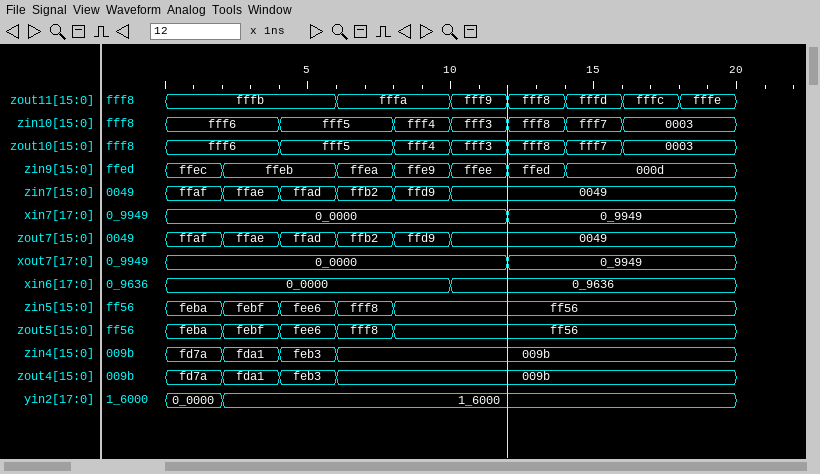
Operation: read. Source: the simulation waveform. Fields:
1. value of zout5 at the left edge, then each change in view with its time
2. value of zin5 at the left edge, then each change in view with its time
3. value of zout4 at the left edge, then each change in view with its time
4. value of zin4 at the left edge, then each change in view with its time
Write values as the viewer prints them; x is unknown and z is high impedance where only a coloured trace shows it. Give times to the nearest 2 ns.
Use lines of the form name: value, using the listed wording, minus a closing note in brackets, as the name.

value of zout5 at the left edge, then each change in view with its time: feba, febf at 2 ns, fee6 at 4 ns, fff8 at 6 ns, ff56 at 8 ns
value of zin5 at the left edge, then each change in view with its time: feba, febf at 2 ns, fee6 at 4 ns, fff8 at 6 ns, ff56 at 8 ns
value of zout4 at the left edge, then each change in view with its time: fd7a, fda1 at 2 ns, feb3 at 4 ns, 009b at 6 ns
value of zin4 at the left edge, then each change in view with its time: fd7a, fda1 at 2 ns, feb3 at 4 ns, 009b at 6 ns
